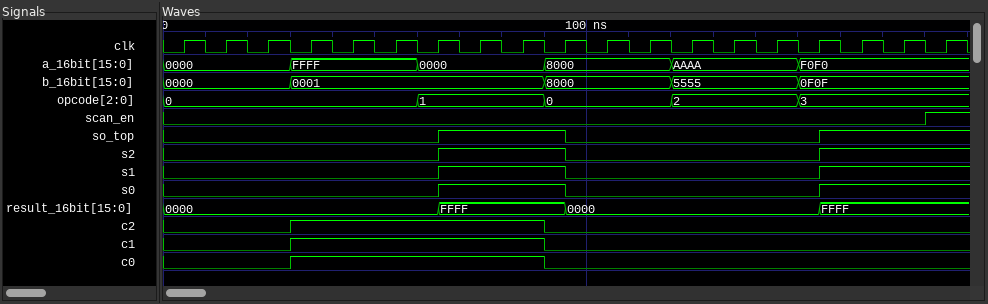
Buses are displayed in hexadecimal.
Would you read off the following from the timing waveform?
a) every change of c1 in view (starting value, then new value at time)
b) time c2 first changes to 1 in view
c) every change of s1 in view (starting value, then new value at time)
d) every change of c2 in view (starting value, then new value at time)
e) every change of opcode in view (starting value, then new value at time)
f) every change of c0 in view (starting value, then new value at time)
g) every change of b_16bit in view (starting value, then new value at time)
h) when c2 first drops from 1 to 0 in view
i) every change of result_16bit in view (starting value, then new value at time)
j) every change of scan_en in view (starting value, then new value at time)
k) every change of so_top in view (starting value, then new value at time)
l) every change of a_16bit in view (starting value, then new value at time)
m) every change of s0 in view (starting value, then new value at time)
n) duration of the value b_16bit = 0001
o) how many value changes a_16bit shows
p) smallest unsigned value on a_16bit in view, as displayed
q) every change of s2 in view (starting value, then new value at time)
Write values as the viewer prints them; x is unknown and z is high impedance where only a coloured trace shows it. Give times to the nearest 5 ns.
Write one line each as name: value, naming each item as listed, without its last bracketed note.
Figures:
every change of c1 in view: 0, 1 at 30 ns, 0 at 90 ns
time c2 first changes to 1 in view: 30 ns
every change of s1 in view: 0, 1 at 65 ns, 0 at 95 ns, 1 at 155 ns
every change of c2 in view: 0, 1 at 30 ns, 0 at 90 ns
every change of opcode in view: 0, 1 at 60 ns, 0 at 90 ns, 2 at 120 ns, 3 at 150 ns
every change of c0 in view: 0, 1 at 30 ns, 0 at 90 ns
every change of b_16bit in view: 0000, 0001 at 30 ns, 8000 at 90 ns, 5555 at 120 ns, 0F0F at 150 ns
when c2 first drops from 1 to 0 in view: 90 ns
every change of result_16bit in view: 0000, FFFF at 65 ns, 0000 at 95 ns, FFFF at 155 ns
every change of scan_en in view: 0, 1 at 180 ns
every change of so_top in view: 0, 1 at 65 ns, 0 at 95 ns, 1 at 155 ns
every change of a_16bit in view: 0000, FFFF at 30 ns, 0000 at 60 ns, 8000 at 90 ns, AAAA at 120 ns, F0F0 at 150 ns
every change of s0 in view: 0, 1 at 65 ns, 0 at 95 ns, 1 at 155 ns
duration of the value b_16bit = 0001: 60 ns
how many value changes a_16bit shows: 5
smallest unsigned value on a_16bit in view, as displayed: 0000
every change of s2 in view: 0, 1 at 65 ns, 0 at 95 ns, 1 at 155 ns
